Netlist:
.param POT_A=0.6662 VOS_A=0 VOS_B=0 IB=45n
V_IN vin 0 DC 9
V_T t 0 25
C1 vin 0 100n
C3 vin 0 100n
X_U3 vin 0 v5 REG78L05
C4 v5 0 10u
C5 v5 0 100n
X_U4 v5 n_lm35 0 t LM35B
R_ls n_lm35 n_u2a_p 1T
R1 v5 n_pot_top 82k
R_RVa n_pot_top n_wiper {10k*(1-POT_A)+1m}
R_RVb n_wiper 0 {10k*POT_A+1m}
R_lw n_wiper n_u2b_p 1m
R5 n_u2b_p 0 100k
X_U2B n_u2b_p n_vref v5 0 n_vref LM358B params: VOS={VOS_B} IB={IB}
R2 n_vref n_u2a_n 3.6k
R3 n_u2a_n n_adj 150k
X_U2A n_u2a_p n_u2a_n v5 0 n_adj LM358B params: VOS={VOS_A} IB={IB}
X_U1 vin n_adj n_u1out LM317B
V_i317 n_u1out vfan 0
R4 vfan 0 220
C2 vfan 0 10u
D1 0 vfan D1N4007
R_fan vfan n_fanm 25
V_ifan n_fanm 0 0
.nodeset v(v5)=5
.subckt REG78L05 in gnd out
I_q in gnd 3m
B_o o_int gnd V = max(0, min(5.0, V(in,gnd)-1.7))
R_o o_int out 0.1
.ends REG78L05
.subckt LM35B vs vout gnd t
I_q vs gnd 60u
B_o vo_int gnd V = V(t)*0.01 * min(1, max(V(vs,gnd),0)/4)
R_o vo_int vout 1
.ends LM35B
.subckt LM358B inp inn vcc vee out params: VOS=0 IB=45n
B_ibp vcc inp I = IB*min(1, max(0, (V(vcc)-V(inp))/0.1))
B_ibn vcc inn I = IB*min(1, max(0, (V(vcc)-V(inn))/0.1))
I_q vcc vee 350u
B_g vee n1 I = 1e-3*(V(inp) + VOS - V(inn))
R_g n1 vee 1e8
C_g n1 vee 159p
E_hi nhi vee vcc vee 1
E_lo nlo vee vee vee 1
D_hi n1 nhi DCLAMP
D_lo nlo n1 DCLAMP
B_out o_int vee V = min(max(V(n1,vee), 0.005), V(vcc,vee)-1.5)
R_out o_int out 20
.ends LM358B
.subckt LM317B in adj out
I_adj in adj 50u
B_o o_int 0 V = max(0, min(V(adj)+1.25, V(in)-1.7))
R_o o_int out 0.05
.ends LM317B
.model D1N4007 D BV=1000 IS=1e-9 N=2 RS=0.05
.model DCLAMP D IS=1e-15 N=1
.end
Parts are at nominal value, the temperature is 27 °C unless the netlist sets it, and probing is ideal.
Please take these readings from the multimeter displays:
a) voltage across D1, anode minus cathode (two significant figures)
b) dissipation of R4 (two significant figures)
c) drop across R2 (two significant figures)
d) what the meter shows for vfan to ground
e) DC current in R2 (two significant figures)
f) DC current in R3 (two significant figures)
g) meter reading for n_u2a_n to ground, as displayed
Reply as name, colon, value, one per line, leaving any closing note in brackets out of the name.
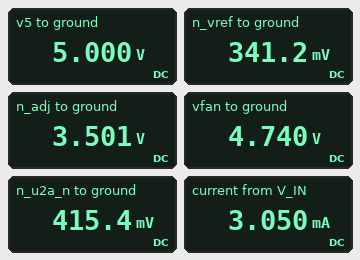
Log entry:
voltage across D1, anode minus cathode: -4.7 V
dissipation of R4: 100 mW
drop across R2: 74 mV
what the meter shows for vfan to ground: 4.740 V
DC current in R2: 21 µA
DC current in R3: 21 µA
meter reading for n_u2a_n to ground, as displayed: 415.4 mV
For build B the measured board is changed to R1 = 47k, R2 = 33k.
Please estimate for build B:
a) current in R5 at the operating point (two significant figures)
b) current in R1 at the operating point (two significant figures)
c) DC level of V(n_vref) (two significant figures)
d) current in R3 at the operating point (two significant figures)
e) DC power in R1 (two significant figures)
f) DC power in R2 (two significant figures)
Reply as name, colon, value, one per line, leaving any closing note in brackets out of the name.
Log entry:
current in R5 at the operating point: 5.5 µA
current in R1 at the operating point: 88 µA
DC level of V(n_vref): 550 mV
current in R3 at the operating point: 16 µA
DC power in R1: 370 µW
DC power in R2: 8.6 µW
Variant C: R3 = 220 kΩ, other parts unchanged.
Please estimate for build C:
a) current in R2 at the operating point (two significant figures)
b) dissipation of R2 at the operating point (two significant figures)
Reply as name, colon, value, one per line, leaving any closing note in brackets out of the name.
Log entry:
current in R2 at the operating point: 14 µA
dissipation of R2 at the operating point: 720 nW
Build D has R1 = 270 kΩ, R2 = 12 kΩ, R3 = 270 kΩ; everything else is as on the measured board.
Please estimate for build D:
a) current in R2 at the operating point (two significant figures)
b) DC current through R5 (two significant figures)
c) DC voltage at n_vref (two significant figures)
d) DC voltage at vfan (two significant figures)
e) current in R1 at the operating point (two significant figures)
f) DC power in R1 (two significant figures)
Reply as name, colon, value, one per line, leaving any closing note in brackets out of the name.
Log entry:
current in R2 at the operating point: 12 µA
DC current through R5: 1.1 µA
DC voltage at n_vref: 110 mV
DC voltage at vfan: 4.7 V
current in R1 at the operating point: 18 µA
DC power in R1: 86 µW
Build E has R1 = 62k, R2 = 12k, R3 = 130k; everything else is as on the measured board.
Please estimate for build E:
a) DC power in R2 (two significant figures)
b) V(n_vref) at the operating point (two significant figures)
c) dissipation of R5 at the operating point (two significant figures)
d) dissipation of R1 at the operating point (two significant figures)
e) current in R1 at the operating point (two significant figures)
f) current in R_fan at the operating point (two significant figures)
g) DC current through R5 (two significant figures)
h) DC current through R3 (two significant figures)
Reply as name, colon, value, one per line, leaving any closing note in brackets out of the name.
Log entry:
DC power in R2: 5.6 µW
V(n_vref) at the operating point: 440 mV
dissipation of R5 at the operating point: 1.9 µW
dissipation of R1 at the operating point: 300 µW
current in R1 at the operating point: 70 µA
current in R_fan at the operating point: 190 mA
DC current through R5: 4.4 µA
DC current through R3: 22 µA
